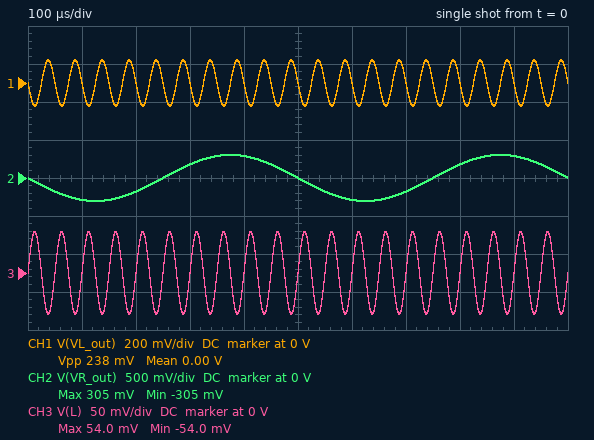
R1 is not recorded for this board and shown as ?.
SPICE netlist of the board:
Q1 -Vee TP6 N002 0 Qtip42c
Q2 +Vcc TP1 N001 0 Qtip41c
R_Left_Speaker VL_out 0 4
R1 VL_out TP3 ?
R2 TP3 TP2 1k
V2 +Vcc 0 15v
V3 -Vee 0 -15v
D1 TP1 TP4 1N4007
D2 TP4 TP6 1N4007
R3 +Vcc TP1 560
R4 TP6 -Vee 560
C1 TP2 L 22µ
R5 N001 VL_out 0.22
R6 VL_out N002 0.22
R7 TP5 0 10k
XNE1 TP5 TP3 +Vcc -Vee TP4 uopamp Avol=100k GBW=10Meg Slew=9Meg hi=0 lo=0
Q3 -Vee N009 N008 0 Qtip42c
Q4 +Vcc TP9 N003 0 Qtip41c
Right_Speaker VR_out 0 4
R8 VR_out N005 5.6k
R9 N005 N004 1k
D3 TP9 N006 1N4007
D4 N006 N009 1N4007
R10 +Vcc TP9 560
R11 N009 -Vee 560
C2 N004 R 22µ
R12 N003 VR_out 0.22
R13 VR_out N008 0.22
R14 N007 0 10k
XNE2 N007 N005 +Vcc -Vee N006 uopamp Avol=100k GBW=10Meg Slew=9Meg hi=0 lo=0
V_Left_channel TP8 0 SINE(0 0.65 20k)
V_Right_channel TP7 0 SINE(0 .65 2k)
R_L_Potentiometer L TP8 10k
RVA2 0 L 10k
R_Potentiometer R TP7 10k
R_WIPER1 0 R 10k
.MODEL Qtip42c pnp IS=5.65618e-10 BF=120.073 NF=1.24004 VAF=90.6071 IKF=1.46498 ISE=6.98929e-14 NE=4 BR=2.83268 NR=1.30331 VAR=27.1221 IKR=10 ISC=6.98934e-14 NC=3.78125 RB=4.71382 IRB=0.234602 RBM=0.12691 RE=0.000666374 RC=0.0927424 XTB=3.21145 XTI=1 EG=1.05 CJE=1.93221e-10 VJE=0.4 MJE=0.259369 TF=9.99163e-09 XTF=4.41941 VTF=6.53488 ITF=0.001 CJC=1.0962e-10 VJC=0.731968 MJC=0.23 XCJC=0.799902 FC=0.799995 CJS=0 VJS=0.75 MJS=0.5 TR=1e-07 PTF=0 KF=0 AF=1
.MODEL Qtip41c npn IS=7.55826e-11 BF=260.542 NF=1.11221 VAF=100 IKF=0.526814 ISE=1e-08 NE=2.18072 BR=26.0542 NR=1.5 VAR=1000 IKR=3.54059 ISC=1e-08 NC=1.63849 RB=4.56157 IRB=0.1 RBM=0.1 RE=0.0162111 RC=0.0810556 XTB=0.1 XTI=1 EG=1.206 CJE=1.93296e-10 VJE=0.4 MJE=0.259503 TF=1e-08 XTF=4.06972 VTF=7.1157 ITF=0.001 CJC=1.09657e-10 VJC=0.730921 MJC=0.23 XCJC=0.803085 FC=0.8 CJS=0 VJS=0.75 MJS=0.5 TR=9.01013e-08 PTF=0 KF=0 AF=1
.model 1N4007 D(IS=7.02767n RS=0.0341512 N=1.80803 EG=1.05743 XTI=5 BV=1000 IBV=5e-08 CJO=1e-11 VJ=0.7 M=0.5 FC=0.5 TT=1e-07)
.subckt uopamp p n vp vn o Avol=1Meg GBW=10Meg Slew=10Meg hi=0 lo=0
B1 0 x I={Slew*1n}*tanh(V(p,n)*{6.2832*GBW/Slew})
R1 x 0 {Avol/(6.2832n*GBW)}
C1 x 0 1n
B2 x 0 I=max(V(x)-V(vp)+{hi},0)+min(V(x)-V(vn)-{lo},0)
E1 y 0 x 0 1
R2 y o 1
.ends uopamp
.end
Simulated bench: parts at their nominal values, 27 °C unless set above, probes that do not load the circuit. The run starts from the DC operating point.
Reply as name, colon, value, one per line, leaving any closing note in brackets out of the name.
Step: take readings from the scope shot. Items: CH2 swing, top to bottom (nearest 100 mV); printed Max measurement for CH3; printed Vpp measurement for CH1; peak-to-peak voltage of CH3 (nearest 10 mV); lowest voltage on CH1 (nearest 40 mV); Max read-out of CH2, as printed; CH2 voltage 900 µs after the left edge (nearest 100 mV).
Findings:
CH2 swing, top to bottom: 600 mV
printed Max measurement for CH3: 54.0 mV
printed Vpp measurement for CH1: 238 mV
peak-to-peak voltage of CH3: 110 mV
lowest voltage on CH1: -120 mV
Max read-out of CH2, as printed: 305 mV
CH2 voltage 900 µs after the left edge: 300 mV
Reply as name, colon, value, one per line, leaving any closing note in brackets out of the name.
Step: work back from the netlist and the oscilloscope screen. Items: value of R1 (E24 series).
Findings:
value of R1: 2.2 kΩ
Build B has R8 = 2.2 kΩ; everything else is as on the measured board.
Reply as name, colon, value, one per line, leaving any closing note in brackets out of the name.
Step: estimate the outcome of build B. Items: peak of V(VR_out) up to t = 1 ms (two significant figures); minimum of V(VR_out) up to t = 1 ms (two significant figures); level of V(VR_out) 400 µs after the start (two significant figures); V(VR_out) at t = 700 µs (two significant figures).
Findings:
peak of V(VR_out) up to t = 1 ms: 120 mV
minimum of V(VR_out) up to t = 1 ms: -120 mV
level of V(VR_out) 400 µs after the start: 110 mV
V(VR_out) at t = 700 µs: -70 mV
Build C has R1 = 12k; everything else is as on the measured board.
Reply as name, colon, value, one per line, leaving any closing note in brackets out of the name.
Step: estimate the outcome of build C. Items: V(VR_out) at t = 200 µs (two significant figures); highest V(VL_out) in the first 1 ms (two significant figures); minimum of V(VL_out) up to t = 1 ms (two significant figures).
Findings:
V(VR_out) at t = 200 µs: -180 mV
highest V(VL_out) in the first 1 ms: 650 mV
minimum of V(VL_out) up to t = 1 ms: -650 mV
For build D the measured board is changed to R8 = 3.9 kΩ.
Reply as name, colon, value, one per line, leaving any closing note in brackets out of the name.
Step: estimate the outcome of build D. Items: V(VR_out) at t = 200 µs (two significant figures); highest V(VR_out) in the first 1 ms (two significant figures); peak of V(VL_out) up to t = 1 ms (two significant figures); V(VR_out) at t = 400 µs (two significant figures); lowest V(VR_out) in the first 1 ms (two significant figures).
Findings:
V(VR_out) at t = 200 µs: -120 mV
highest V(VR_out) in the first 1 ms: 210 mV
peak of V(VL_out) up to t = 1 ms: 120 mV
V(VR_out) at t = 400 µs: 200 mV
lowest V(VR_out) in the first 1 ms: -210 mV
